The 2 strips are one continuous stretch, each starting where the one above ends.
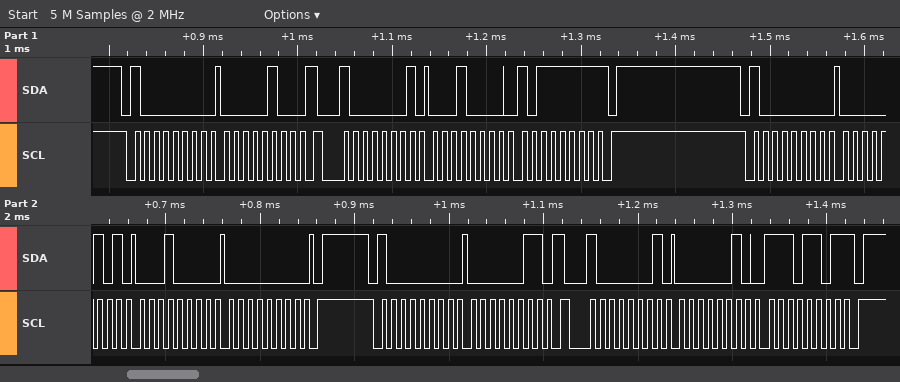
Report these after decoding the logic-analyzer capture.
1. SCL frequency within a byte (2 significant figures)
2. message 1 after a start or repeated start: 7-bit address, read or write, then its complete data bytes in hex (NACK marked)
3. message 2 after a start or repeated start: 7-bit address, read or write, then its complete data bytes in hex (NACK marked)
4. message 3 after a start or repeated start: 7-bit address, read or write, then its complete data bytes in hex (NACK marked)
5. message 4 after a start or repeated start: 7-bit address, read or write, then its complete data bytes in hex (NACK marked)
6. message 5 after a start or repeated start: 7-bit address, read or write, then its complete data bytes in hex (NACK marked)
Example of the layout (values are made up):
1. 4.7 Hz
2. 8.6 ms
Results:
1. 100 kHz
2. 0x40 write: 04
3. 0x40 read: 10 BF NACK
4. 0x40 write: 05 10 00
5. 0x40 write: 03
6. 0x40 read: 02 ED NACK
